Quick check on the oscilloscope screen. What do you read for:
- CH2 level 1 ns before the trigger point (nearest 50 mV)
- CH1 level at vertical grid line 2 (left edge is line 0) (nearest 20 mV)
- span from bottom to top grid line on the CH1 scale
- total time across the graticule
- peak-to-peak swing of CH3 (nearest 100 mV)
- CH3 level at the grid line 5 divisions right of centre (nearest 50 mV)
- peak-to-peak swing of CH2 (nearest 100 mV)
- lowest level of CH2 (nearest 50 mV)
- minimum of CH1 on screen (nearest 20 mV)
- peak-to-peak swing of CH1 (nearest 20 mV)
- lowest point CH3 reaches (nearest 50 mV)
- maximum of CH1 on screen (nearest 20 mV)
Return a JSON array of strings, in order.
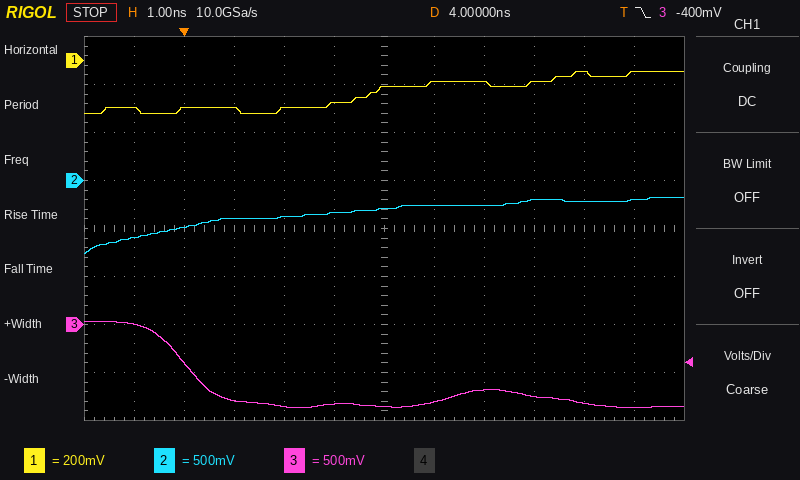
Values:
["-600 mV", "-200 mV", "1.6 V", "12 ns", "900 mV", "-850 mV", "600 mV", "-750 mV", "-220 mV", "180 mV", "-850 mV", "-40 mV"]
